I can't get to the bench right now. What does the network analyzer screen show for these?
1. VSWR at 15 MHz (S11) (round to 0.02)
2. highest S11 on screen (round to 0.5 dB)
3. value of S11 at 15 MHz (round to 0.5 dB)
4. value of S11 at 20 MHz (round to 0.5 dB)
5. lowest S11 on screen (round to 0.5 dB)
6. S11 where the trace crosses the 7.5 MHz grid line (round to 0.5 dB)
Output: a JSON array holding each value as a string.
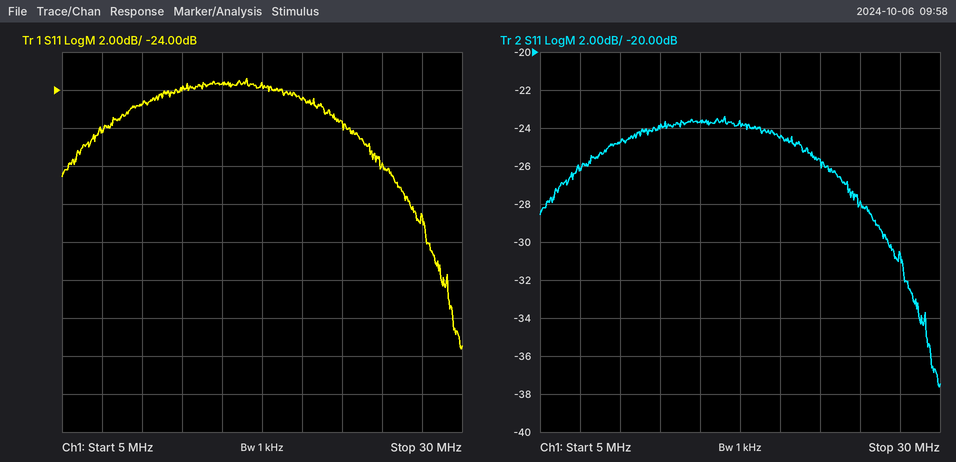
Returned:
["1.14", "-23.5 dB", "-23.5 dB", "-24.5 dB", "-37.5 dB", "-26.0 dB"]
